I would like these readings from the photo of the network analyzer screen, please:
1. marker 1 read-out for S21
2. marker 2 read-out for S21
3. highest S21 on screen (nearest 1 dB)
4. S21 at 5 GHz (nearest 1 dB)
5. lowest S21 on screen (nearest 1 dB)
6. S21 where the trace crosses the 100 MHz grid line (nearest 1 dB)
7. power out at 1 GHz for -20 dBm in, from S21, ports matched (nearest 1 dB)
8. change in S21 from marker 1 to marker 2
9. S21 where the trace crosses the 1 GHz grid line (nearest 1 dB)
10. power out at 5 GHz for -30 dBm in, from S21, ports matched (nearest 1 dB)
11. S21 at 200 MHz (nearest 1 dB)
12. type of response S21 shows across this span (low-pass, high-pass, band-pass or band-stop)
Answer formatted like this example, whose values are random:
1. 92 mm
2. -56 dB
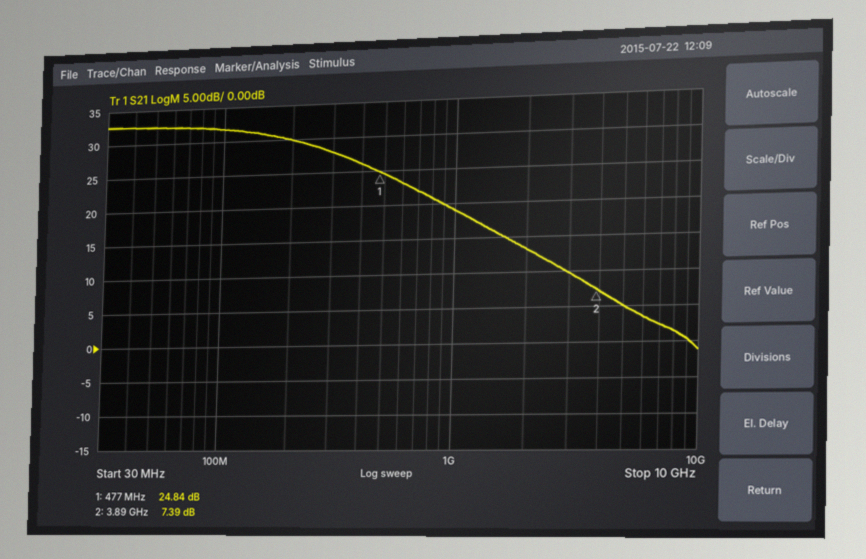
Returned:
1. 24.84 dB
2. 7.39 dB
3. 33 dB
4. 5 dB
5. -1 dB
6. 32 dB
7. -1 dBm
8. -17.45 dB
9. 19 dB
10. -25 dBm
11. 30 dB
12. low-pass
